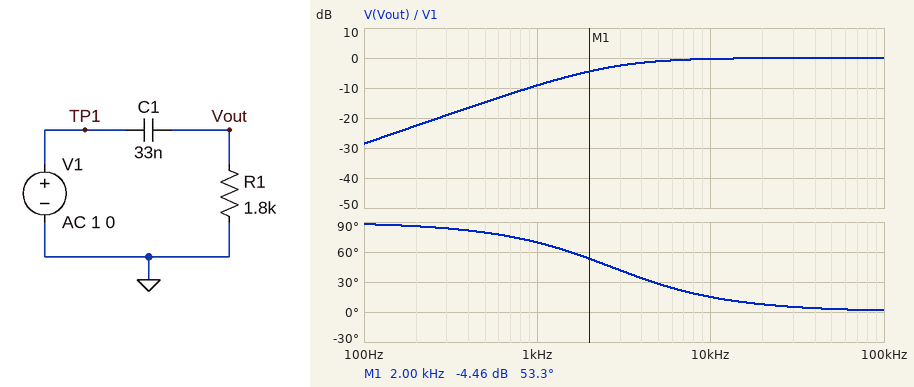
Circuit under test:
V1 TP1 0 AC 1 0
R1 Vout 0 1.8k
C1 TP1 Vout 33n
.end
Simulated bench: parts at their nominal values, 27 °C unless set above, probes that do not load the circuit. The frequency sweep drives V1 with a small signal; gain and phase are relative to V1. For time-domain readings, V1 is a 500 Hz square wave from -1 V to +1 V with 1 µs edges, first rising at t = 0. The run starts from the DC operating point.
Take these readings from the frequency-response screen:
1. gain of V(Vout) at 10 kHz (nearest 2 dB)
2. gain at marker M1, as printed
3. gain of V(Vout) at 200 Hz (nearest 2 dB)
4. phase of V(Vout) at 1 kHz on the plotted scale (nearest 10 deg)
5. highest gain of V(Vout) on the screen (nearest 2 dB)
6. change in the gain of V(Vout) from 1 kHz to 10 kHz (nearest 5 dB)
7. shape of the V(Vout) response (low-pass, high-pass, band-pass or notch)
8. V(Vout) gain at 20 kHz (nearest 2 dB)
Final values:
0 dB
-4.46 dB
-22 dB
70 deg
0 dB
10 dB
high-pass
0 dB
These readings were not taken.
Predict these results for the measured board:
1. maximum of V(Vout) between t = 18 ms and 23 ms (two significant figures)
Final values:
2.0 V
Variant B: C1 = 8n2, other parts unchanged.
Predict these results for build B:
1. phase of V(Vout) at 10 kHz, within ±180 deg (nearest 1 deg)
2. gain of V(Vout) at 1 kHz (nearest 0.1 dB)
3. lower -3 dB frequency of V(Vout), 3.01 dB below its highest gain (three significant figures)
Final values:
47 deg
-20.7 dB
10.8 kHz
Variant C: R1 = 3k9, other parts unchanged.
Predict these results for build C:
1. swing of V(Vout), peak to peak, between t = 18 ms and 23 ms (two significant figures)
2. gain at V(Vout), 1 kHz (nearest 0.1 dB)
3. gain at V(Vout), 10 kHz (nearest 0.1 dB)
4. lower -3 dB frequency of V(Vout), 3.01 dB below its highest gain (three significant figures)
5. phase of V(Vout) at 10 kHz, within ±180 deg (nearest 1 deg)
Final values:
4.0 V
-4.0 dB
-0.1 dB
1.24 kHz
7 deg
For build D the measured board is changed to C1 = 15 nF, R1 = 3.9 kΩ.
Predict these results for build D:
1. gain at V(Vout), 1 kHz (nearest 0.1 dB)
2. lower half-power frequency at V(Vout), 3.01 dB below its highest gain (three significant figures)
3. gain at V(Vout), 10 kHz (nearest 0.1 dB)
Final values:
-9.2 dB
2.72 kHz
-0.3 dB
